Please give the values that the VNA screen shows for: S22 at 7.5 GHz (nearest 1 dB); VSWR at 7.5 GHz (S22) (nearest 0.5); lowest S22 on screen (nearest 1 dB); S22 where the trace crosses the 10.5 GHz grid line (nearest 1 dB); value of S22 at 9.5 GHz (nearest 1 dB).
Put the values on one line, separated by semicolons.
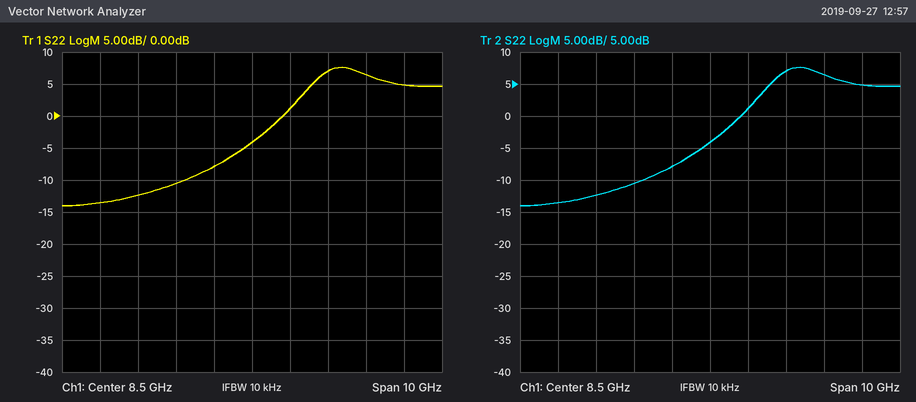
-8 dB; 2.5; -14 dB; 7 dB; 1 dB
